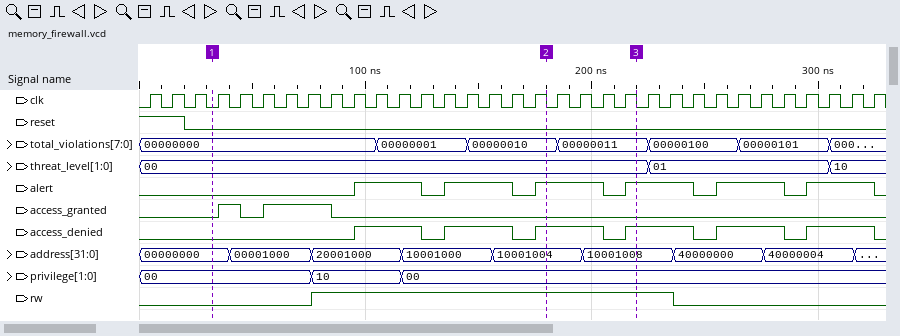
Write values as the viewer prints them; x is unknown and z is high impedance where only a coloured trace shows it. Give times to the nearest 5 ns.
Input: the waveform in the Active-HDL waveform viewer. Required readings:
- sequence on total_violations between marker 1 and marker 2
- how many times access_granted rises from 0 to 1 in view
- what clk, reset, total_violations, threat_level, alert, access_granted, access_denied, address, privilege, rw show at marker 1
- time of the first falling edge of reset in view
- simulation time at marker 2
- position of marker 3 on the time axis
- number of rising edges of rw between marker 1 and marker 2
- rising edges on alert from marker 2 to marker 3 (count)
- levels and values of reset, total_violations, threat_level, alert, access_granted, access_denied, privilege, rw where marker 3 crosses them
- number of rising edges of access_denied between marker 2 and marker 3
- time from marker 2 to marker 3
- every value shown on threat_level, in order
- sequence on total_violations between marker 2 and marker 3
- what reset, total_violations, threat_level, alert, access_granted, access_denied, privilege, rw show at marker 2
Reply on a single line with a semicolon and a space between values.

00000000, 00000001, 00000010; 2; clk=0, reset=0, total_violations=00000000, threat_level=00, alert=0, access_granted=0, access_denied=0, address=00000000, privilege=00, rw=0; 20 ns; 180 ns; 220 ns; 1; 1; reset=0, total_violations=00000011, threat_level=00, alert=1, access_granted=0, access_denied=1, privilege=00, rw=1; 1; 40 ns; 00, 01, 10; 00000010, 00000011; reset=0, total_violations=00000010, threat_level=00, alert=1, access_granted=0, access_denied=1, privilege=00, rw=1
